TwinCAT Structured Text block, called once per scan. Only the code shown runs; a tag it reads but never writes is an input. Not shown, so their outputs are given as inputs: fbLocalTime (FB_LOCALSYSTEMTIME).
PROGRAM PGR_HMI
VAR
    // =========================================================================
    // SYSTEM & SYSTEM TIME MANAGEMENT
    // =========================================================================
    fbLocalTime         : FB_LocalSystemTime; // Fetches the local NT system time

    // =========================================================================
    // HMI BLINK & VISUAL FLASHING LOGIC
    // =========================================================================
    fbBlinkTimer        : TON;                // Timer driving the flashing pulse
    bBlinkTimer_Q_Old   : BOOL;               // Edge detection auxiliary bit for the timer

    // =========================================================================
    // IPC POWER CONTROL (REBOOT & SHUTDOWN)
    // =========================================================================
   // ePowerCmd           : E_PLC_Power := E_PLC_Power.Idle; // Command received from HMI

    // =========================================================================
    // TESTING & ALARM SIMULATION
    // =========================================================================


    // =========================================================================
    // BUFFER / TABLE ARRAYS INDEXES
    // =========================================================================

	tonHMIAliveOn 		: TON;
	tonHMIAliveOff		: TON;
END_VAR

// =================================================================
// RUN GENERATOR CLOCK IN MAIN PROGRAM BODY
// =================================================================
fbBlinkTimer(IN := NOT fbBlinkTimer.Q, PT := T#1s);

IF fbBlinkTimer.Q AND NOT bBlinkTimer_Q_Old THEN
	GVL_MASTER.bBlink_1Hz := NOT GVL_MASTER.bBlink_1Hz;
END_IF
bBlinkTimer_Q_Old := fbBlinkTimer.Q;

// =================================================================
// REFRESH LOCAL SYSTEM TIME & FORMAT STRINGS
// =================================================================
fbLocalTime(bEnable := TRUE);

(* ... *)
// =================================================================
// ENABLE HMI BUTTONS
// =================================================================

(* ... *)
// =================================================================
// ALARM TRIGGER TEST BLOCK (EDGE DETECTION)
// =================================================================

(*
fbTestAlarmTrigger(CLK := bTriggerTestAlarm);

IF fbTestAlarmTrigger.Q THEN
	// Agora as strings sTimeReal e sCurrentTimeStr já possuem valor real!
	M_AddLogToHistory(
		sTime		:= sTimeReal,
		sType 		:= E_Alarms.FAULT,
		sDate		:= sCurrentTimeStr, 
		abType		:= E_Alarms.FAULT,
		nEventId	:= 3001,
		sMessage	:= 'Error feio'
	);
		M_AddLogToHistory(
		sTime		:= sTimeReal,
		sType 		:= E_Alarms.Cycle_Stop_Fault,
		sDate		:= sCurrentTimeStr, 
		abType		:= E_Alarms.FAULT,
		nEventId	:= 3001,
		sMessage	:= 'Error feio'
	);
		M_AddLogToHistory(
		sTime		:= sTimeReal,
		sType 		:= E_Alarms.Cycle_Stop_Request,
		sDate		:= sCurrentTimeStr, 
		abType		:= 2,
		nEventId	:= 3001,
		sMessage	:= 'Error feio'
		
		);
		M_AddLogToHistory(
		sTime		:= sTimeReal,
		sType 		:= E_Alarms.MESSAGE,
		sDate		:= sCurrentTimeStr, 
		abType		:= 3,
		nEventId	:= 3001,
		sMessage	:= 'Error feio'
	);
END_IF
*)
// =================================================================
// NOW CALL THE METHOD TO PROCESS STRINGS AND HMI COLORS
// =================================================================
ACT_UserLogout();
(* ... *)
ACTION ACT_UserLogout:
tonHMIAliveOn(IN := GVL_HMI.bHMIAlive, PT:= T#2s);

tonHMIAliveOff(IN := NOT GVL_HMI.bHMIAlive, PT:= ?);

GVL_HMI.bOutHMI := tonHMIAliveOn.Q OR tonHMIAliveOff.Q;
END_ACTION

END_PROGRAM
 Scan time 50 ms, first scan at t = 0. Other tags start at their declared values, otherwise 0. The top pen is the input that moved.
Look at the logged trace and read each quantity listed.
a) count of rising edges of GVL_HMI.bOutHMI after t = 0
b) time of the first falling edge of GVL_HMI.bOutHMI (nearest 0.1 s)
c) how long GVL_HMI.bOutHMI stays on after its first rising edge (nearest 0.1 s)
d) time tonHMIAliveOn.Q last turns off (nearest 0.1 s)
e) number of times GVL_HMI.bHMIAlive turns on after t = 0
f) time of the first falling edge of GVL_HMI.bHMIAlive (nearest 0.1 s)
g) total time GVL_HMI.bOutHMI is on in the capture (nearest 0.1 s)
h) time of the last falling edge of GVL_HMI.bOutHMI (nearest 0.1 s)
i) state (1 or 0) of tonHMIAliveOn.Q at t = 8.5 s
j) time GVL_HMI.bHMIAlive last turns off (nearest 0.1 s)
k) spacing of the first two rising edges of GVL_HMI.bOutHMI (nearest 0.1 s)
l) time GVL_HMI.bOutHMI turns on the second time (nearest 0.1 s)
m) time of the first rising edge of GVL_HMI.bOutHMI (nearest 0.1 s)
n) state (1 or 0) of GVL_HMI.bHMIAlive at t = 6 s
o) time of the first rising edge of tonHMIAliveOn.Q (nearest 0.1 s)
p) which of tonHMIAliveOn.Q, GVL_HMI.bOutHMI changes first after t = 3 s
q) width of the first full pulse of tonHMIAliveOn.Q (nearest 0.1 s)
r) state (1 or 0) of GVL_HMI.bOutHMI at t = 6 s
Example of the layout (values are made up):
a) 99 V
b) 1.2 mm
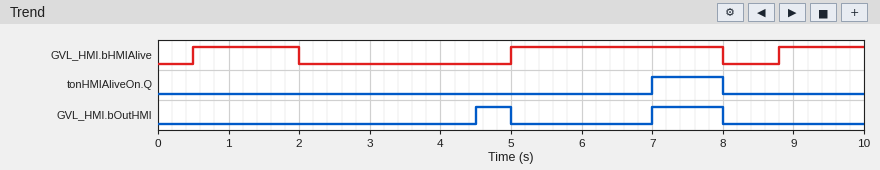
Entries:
a) 2
b) 5.0 s
c) 0.5 s
d) 8.0 s
e) 3
f) 2.0 s
g) 1.5 s
h) 8.0 s
i) 0
j) 8.0 s
k) 2.5 s
l) 7.0 s
m) 4.5 s
n) 1
o) 7.0 s
p) GVL_HMI.bOutHMI
q) 1.0 s
r) 0
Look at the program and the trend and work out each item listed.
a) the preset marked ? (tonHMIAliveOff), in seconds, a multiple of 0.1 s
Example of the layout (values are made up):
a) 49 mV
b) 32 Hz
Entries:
a) 2.5 s
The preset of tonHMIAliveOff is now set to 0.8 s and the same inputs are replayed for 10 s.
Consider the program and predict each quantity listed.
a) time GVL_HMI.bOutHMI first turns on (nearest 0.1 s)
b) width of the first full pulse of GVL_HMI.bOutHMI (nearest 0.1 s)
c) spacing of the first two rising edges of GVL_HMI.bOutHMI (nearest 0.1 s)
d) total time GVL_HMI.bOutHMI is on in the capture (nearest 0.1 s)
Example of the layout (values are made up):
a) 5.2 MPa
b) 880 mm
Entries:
a) 2.8 s
b) 2.2 s
c) 4.2 s
d) 3.2 s
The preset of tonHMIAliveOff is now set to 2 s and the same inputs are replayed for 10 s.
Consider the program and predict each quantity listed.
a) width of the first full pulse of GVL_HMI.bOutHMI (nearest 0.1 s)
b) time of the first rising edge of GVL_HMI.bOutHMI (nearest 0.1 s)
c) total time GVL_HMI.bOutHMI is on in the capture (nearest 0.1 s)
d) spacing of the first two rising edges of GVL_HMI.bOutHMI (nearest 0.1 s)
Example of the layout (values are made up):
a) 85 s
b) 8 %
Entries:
a) 1.0 s
b) 4.0 s
c) 2.0 s
d) 3.0 s
